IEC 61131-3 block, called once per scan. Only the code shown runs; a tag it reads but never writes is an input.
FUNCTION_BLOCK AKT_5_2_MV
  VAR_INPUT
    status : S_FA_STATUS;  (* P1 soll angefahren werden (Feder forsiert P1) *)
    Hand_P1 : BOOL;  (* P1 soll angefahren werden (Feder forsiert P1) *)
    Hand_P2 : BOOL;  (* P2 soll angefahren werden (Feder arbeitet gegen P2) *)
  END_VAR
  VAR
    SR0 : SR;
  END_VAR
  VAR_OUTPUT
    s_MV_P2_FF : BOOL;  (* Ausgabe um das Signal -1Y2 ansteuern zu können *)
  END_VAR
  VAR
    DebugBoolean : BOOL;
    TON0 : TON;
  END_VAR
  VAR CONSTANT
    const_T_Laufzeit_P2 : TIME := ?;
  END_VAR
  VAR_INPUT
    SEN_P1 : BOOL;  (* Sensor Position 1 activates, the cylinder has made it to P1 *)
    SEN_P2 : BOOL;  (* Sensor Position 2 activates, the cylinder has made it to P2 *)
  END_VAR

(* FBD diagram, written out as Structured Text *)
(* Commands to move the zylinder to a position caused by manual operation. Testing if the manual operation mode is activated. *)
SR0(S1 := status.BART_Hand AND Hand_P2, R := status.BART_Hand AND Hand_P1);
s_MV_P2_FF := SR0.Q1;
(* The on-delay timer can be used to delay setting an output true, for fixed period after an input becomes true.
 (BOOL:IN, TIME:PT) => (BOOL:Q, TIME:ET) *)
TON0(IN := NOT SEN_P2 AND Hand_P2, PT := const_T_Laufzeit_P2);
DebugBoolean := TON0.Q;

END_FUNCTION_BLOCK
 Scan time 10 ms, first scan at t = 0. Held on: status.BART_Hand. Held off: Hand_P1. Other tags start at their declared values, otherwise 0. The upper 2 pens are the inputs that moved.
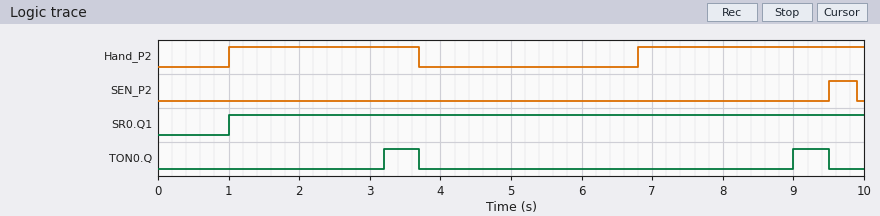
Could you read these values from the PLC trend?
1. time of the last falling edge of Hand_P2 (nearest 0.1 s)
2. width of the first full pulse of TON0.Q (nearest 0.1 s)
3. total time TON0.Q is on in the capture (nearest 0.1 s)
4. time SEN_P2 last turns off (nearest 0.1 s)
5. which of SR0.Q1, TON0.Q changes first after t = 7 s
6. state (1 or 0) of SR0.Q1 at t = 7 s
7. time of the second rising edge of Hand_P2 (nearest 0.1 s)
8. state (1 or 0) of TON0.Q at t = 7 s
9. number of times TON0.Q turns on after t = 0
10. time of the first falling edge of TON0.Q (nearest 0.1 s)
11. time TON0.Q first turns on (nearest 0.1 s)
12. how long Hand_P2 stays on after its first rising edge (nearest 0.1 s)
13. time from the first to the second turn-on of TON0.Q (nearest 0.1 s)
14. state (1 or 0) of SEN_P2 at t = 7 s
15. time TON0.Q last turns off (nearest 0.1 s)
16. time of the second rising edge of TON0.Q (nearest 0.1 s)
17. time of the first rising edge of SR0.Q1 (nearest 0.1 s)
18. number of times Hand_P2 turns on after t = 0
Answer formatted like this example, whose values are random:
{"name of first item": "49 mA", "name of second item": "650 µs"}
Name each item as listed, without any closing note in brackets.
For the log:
{"time of the last falling edge of Hand_P2": "3.7 s", "width of the first full pulse of TON0.Q": "0.5 s", "total time TON0.Q is on in the capture": "1.0 s", "time SEN_P2 last turns off": "9.9 s", "which of SR0.Q1, TON0.Q changes first after t = 7 s": "TON0.Q", "state (1 or 0) of SR0.Q1 at t = 7 s": "1", "time of the second rising edge of Hand_P2": "6.8 s", "state (1 or 0) of TON0.Q at t = 7 s": "0", "number of times TON0.Q turns on after t = 0": "2", "time of the first falling edge of TON0.Q": "3.7 s", "time TON0.Q first turns on": "3.2 s", "how long Hand_P2 stays on after its first rising edge": "2.7 s", "time from the first to the second turn-on of TON0.Q": "5.8 s", "state (1 or 0) of SEN_P2 at t = 7 s": "0", "time TON0.Q last turns off": "9.5 s", "time of the second rising edge of TON0.Q": "9.0 s", "time of the first rising edge of SR0.Q1": "1.0 s", "number of times Hand_P2 turns on after t = 0": "2"}
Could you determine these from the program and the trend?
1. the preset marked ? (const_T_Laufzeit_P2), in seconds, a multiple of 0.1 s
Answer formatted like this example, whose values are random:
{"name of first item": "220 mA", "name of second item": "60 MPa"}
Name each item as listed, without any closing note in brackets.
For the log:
{"the preset marked ? (const_T_Laufzeit_P2), in seconds, a multiple of 0.1 s": "2.2 s"}
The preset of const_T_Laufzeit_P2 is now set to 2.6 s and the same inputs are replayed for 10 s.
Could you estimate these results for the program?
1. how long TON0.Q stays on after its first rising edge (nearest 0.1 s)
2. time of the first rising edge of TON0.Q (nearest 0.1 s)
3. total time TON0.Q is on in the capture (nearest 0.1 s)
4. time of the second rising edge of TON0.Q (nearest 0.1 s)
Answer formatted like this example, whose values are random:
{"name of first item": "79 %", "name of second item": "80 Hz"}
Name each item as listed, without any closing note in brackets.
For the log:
{"how long TON0.Q stays on after its first rising edge": "0.1 s", "time of the first rising edge of TON0.Q": "3.6 s", "total time TON0.Q is on in the capture": "0.2 s", "time of the second rising edge of TON0.Q": "9.4 s"}
